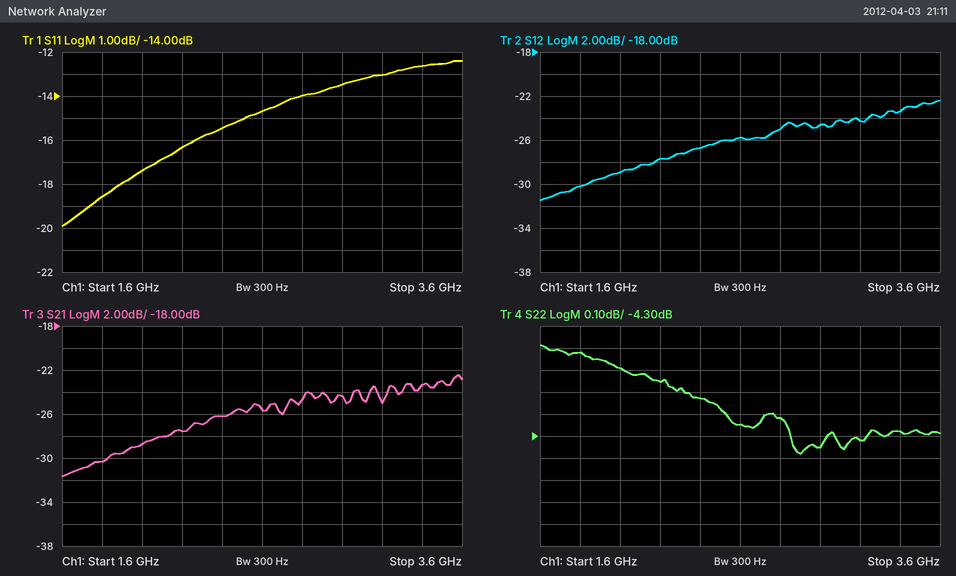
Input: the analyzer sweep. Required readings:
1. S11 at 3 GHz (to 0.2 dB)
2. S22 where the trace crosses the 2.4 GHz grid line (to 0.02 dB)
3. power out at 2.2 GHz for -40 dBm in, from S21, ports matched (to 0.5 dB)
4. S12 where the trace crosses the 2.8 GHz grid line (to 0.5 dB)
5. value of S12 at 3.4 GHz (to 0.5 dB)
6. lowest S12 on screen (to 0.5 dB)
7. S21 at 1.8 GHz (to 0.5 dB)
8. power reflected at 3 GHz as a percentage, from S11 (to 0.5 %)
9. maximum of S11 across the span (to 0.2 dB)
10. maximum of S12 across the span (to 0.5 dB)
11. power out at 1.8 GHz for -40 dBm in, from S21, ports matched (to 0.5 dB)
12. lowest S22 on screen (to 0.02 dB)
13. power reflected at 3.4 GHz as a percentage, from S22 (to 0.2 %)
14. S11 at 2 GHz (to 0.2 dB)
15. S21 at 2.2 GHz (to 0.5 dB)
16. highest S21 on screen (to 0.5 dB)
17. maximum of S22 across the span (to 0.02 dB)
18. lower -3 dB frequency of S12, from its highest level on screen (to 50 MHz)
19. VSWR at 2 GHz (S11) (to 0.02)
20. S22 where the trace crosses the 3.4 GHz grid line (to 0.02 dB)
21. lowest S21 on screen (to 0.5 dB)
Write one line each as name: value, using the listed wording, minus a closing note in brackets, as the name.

S11 at 3 GHz: -13.4 dB
S22 where the trace crosses the 2.4 GHz grid line: -4.12 dB
power out at 2.2 GHz for -40 dBm in, from S21, ports matched: -67.5 dBm
S12 where the trace crosses the 2.8 GHz grid line: -25.0 dB
value of S12 at 3.4 GHz: -23.5 dB
lowest S12 on screen: -31.5 dB
S21 at 1.8 GHz: -30.5 dB
power reflected at 3 GHz as a percentage, from S11: 4.5 %
maximum of S11 across the span: -12.4 dB
maximum of S12 across the span: -22.5 dB
power out at 1.8 GHz for -40 dBm in, from S21, ports matched: -70.5 dBm
lowest S22 on screen: -4.38 dB
power reflected at 3.4 GHz as a percentage, from S22: 37.4 %
S11 at 2 GHz: -17.4 dB
S21 at 2.2 GHz: -27.5 dB
highest S21 on screen: -22.5 dB
maximum of S22 across the span: -3.88 dB
lower -3 dB frequency of S12, from its highest level on screen: 2.75 GHz
VSWR at 2 GHz (S11): 1.32
S22 where the trace crosses the 3.4 GHz grid line: -4.28 dB
lowest S21 on screen: -31.5 dB
